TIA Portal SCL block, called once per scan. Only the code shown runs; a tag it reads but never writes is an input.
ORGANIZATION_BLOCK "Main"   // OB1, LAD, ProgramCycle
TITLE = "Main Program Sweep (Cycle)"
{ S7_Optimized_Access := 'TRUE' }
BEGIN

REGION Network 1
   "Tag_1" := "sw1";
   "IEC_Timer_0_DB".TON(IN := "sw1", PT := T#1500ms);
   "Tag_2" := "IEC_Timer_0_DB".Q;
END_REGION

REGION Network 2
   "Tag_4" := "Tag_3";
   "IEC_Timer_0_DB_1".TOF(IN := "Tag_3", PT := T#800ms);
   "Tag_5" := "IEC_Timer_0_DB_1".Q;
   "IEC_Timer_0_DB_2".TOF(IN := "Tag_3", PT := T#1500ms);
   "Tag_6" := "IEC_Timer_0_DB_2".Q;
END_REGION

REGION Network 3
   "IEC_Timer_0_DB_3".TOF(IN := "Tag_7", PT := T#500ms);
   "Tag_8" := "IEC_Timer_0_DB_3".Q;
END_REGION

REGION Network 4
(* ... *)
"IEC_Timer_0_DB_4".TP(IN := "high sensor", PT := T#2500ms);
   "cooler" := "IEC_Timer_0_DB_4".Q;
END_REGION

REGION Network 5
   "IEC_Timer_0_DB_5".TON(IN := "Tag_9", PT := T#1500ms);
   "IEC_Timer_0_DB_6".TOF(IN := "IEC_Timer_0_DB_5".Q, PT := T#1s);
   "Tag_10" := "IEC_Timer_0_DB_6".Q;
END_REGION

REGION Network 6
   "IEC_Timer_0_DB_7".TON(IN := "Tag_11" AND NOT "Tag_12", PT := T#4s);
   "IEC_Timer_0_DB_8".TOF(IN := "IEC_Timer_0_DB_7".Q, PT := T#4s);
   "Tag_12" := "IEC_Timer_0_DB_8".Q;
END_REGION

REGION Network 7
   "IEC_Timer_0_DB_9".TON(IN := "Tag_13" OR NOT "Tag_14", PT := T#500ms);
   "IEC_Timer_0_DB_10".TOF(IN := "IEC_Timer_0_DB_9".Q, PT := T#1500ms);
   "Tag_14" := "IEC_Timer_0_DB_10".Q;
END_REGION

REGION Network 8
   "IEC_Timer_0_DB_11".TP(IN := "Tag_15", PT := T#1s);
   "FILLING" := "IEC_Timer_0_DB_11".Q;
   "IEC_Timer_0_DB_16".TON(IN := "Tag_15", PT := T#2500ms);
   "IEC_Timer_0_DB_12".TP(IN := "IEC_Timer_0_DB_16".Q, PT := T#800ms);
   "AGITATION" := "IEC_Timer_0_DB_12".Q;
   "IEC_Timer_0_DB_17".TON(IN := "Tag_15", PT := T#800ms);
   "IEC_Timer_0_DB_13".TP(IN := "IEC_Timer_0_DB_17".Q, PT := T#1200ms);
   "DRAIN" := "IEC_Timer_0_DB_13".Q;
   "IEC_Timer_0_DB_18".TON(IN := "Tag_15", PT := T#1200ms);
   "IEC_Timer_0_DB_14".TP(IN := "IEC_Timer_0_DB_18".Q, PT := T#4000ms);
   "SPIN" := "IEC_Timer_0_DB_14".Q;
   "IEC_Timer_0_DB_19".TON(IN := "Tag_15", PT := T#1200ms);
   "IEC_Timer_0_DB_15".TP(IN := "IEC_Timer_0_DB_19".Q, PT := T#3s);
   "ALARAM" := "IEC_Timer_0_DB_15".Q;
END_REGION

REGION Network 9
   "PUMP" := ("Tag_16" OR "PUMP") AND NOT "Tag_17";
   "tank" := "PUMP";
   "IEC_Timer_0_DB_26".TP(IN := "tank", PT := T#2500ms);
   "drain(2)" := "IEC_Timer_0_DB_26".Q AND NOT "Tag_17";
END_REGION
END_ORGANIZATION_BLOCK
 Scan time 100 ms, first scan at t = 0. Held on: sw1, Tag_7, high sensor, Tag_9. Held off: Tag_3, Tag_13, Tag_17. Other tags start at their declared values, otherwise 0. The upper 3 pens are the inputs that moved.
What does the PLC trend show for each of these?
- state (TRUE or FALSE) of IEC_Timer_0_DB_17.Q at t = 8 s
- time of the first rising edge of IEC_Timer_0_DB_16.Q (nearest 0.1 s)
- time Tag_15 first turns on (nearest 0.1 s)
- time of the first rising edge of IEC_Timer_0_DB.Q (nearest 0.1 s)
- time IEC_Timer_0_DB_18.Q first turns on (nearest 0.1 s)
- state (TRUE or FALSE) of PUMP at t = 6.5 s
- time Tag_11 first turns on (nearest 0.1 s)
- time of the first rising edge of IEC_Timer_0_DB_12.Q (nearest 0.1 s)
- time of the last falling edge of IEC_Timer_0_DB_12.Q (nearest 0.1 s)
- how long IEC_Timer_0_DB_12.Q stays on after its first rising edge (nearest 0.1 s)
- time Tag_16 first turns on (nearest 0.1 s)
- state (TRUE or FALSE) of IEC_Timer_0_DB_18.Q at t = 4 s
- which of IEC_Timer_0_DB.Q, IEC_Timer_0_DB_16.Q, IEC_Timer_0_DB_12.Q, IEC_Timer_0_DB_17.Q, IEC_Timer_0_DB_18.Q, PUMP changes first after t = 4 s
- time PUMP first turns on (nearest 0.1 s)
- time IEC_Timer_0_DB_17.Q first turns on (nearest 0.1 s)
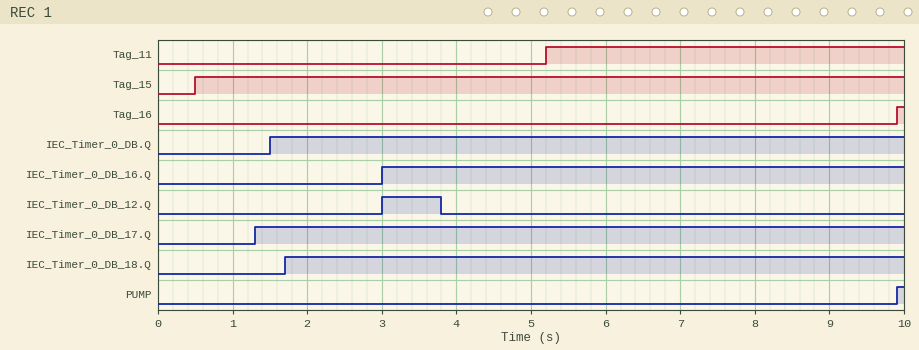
TRUE
3.0 s
0.5 s
1.5 s
1.7 s
FALSE
5.2 s
3.0 s
3.8 s
0.8 s
9.9 s
TRUE
PUMP
9.9 s
1.3 s
